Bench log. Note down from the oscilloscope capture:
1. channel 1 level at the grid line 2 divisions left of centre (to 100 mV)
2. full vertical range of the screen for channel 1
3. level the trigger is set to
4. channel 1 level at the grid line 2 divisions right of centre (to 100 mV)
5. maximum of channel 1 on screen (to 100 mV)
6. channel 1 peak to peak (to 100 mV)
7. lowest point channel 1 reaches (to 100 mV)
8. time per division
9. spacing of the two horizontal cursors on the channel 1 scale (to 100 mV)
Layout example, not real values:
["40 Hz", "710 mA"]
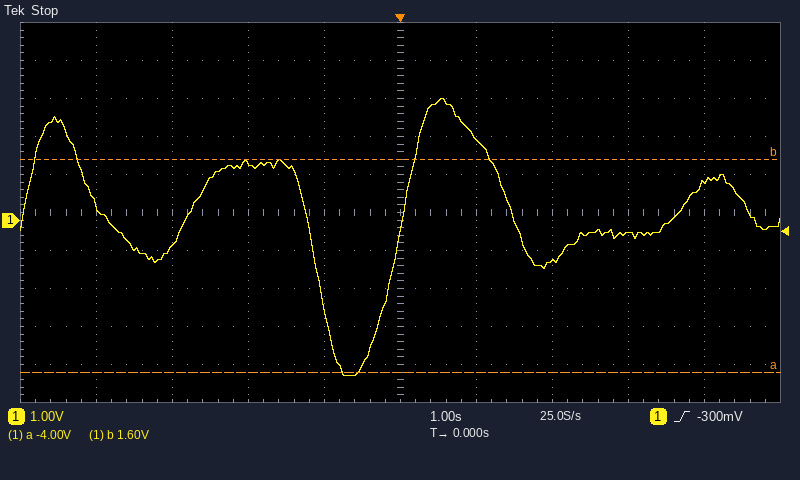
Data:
["1.5 V", "10 V", "-300 mV", "-1.1 V", "3.2 V", "7.3 V", "-4.1 V", "1 s", "5.6 V"]
